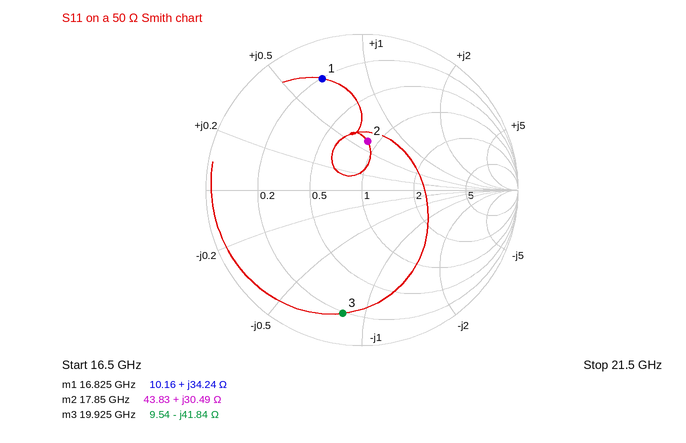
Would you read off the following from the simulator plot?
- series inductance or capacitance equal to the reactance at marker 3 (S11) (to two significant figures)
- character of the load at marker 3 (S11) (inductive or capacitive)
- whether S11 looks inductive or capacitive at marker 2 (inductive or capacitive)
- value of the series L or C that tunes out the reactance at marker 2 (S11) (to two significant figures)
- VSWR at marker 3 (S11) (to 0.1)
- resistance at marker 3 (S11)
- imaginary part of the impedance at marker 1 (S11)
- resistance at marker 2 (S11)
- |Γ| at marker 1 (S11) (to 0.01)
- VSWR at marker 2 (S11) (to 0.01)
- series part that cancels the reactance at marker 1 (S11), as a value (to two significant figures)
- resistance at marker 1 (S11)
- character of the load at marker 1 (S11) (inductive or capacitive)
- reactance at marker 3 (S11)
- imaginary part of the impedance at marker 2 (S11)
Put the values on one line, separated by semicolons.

190 fF; capacitive; inductive; 290 fF; 9.0; 9.54 Ω; +34.24 Ω; 43.83 Ω; 0.76; 1.92; 280 fF; 10.16 Ω; inductive; -41.84 Ω; +30.49 Ω
